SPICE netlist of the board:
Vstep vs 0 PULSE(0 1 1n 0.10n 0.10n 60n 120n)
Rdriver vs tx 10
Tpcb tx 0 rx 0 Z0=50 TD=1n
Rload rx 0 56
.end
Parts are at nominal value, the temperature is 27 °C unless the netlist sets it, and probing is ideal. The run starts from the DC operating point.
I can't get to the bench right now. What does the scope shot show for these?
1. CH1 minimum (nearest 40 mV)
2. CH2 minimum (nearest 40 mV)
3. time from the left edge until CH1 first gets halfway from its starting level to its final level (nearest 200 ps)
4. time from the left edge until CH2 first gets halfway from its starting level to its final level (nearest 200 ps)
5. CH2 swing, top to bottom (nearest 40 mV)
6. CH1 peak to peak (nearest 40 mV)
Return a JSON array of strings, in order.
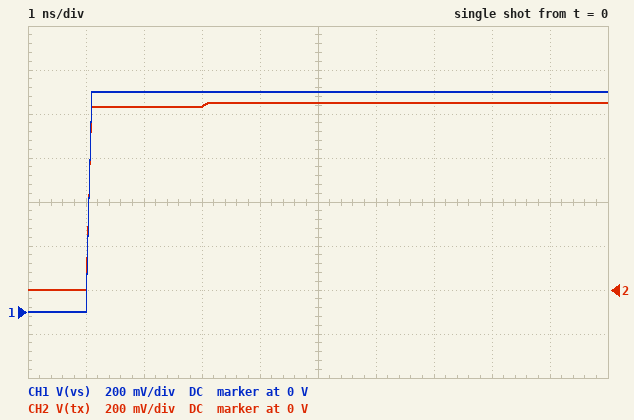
["0 V", "0 V", "1.0 ns", "1.0 ns", "840 mV", "1.00 V"]
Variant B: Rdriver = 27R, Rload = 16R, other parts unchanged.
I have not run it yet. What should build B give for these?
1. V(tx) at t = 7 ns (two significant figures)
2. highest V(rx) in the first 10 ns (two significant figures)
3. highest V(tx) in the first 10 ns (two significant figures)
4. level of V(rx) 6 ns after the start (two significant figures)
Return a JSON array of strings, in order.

["380 mV", "370 mV", "650 mV", "360 mV"]
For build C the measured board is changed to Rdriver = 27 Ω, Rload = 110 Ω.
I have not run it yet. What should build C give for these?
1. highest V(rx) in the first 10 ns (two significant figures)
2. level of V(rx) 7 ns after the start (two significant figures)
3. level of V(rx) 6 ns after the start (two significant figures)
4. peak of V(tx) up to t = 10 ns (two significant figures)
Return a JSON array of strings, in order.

["890 mV", "800 mV", "790 mV", "820 mV"]
